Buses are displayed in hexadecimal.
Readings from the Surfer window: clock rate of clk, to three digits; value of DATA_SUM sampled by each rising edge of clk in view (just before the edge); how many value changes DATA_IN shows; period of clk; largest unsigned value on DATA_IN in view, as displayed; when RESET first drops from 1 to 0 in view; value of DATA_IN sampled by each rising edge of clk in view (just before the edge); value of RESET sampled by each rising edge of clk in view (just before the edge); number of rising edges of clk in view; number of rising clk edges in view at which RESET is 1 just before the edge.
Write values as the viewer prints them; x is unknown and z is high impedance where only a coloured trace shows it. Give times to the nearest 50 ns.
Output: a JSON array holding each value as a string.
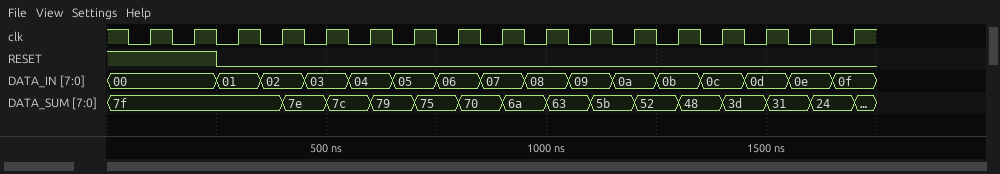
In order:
["10.0 MHz", "7f, 7f, 7f, 7f, 7e, 7c, 79, 75, 70, 6a, 63, 5b, 52, 48, 3d, 31, 24", "15", "100 ns", "0f", "250 ns", "00, 00, 01, 02, 03, 04, 05, 06, 07, 08, 09, 0a, 0b, 0c, 0d, 0e, 0f", "1 1 0 0 0 0 0 0 0 0 0 0 0 0 0 0 0", "17", "2"]
